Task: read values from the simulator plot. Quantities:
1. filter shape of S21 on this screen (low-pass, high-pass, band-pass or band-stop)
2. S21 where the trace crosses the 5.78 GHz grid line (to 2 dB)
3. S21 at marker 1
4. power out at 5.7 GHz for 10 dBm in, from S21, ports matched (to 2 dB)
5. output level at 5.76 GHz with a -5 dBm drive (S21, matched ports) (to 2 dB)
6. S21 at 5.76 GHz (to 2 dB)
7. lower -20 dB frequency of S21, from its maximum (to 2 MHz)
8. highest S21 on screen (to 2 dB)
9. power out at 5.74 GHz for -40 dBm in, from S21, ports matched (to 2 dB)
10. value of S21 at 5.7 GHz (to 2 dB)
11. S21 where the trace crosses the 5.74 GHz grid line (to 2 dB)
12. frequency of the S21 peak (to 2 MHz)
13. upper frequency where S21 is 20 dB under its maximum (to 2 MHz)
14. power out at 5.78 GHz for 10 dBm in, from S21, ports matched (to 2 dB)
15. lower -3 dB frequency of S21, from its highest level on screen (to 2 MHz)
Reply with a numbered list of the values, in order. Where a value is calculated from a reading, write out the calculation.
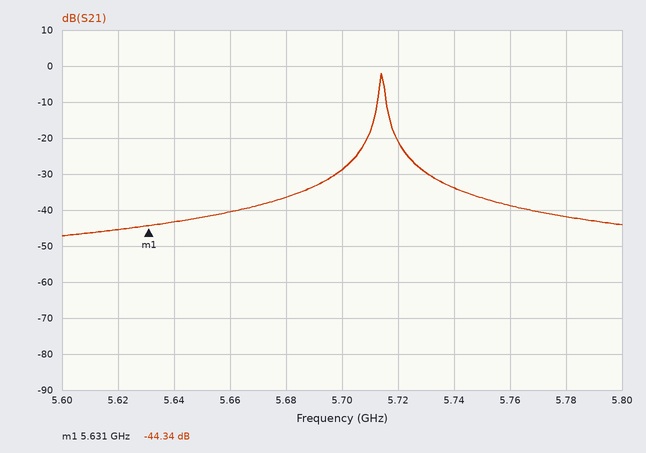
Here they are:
1. band-pass
2. -42 dB
3. -44.34 dB
4. 10 dBm + (-28 dB) = -18 dBm
5. -5 dBm + (-38 dB) = -44 dBm
6. -38 dB
7. 5.708 GHz
8. -2 dB
9. -40 dBm + (-34 dB) = -74 dBm
10. -28 dB
11. -34 dB
12. 5.714 GHz
13. 5.720 GHz
14. 10 dBm + (-42 dB) = -32 dBm
15. 5.714 GHz
